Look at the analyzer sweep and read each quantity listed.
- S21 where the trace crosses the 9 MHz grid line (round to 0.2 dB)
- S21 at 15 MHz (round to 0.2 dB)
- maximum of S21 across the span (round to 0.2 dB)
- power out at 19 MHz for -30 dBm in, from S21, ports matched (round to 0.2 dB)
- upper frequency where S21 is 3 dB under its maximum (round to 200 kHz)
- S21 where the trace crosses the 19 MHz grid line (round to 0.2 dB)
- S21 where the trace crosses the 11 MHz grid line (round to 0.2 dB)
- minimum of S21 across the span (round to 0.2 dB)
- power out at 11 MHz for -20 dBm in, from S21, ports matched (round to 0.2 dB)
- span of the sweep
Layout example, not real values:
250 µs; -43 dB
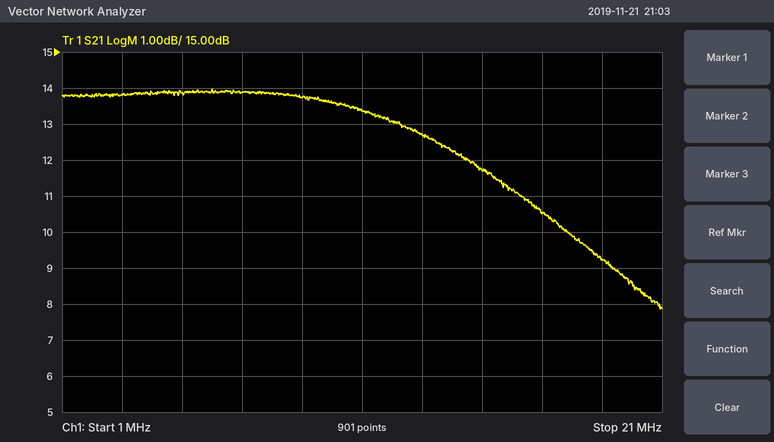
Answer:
13.8 dB; 11.8 dB; 14.0 dB; -20.8 dBm; 16.4 MHz; 9.2 dB; 13.4 dB; 7.8 dB; -6.6 dBm; 20 MHz
